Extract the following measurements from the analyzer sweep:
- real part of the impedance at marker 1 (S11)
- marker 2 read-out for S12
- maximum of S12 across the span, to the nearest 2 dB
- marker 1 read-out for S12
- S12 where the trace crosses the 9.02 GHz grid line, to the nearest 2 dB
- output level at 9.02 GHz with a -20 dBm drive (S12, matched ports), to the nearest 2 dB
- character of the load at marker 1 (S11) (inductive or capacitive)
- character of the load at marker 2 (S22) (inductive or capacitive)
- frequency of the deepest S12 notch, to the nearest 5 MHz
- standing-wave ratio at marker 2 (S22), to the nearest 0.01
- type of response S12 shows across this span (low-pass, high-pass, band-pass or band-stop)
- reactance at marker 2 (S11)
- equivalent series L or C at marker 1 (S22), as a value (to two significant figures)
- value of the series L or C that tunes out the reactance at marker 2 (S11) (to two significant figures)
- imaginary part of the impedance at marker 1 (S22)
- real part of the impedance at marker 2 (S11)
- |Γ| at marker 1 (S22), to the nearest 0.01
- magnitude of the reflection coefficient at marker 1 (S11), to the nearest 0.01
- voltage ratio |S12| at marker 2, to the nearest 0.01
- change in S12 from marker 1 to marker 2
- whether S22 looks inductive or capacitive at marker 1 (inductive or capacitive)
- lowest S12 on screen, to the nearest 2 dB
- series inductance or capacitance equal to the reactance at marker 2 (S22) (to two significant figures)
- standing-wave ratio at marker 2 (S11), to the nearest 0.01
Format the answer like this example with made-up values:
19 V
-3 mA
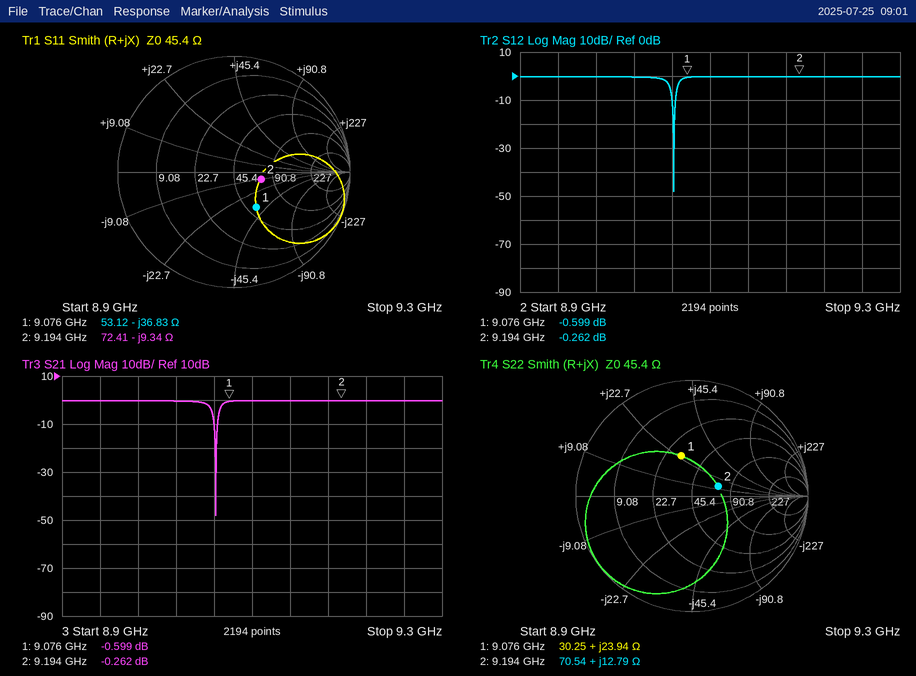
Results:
53.12 Ω
-0.262 dB
0 dB
-0.599 dB
0 dB
-20 dBm
capacitive
inductive
9.060 GHz
1.64
band-stop
-9.34 Ω
420 pH
160 pH
+23.94 Ω
72.41 Ω
0.36
0.36
0.97
0.337 dB
inductive
-48 dB
220 pH
1.64
